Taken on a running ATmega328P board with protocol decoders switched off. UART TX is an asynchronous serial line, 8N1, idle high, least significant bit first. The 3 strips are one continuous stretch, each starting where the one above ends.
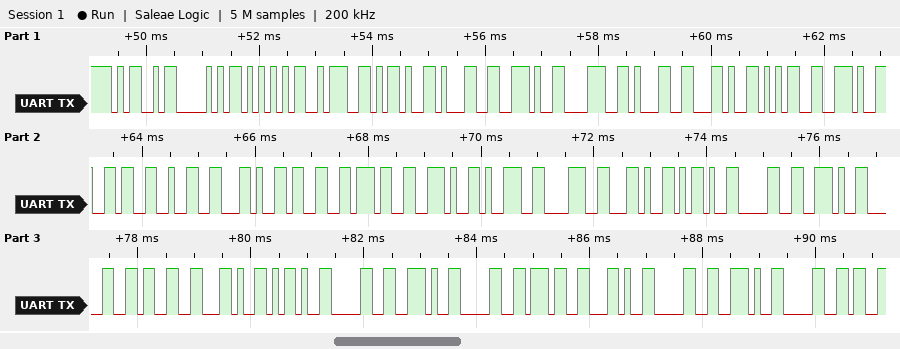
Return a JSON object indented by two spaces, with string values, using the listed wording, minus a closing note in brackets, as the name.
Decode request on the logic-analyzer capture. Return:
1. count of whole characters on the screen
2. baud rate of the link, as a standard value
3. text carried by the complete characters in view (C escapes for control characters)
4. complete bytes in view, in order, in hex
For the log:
{
  "count of whole characters on the screen": "36",
  "baud rate of the link, as a standard value": "9600 baud",
  "text carried by the complete characters in view": "\"MPU:-1.81,5.62,37.98,-0.03,-0.07,0.0\"",
  "complete bytes in view, in order, in hex": "0x4D 0x50 0x55 0x3A 0x2D 0x31 0x2E 0x38 0x31 0x2C 0x35 0x2E 0x36 0x32 0x2C 0x33 0x37 0x2E 0x39 0x38 0x2C 0x2D 0x30 0x2E 0x30 0x33 0x2C 0x2D 0x30 0x2E 0x30 0x37 0x2C 0x30 0x2E 0x30"
}
